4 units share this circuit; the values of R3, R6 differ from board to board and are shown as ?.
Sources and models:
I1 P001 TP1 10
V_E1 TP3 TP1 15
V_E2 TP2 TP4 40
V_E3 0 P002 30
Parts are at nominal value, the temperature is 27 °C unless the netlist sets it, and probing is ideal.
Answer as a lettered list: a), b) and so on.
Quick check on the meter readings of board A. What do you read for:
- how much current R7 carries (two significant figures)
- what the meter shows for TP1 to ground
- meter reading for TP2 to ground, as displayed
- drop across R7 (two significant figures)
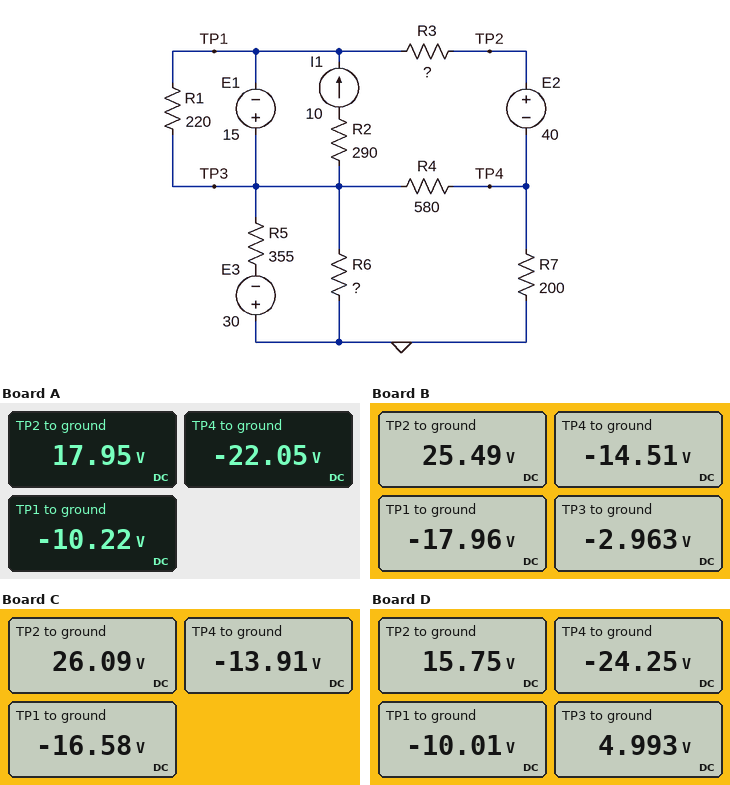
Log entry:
a) 110 mA
b) -10.22 V
c) 17.95 V
d) 22 V
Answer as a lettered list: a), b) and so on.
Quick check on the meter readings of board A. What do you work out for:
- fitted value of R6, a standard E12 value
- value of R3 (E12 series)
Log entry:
a) 390 Ω
b) 180 Ω
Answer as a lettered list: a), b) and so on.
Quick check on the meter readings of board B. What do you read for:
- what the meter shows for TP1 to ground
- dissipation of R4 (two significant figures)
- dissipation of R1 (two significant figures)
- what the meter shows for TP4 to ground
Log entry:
a) -17.96 V
b) 230 mW
c) 1.0 W
d) -14.51 V
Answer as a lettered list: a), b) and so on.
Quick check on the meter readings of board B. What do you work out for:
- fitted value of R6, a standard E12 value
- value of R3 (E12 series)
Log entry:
a) 820 Ω
b) 470 Ω
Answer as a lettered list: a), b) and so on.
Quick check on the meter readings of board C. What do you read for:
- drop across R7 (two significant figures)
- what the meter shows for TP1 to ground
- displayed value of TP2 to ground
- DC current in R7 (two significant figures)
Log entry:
a) 14 V
b) -16.58 V
c) 26.09 V
d) 70 mA
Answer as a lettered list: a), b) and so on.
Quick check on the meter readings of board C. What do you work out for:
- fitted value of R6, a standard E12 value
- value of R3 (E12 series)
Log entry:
a) 150 Ω
b) 470 Ω
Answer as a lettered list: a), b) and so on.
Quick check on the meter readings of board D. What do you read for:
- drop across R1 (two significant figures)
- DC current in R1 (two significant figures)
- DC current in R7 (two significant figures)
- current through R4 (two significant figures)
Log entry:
a) 15 V
b) 68 mA
c) 120 mA
d) 50 mA
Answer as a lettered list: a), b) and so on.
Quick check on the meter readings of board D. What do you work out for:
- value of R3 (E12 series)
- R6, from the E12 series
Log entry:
a) 150 Ω
b) 220 Ω
